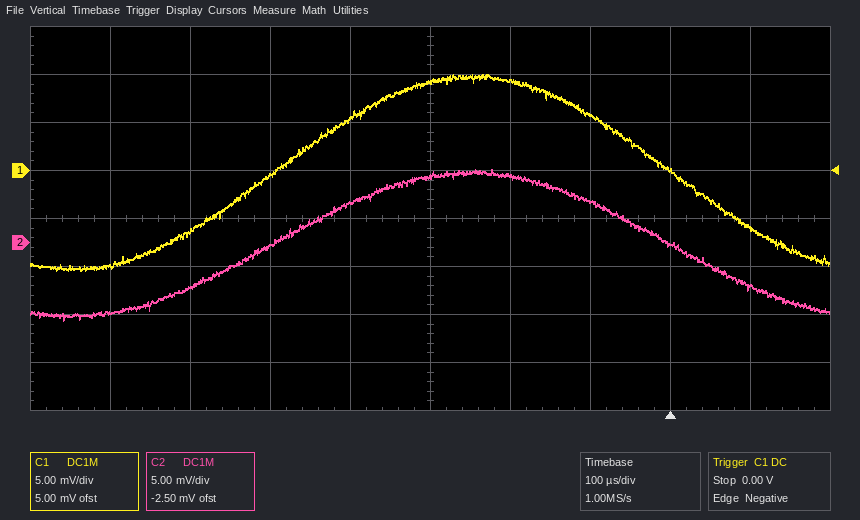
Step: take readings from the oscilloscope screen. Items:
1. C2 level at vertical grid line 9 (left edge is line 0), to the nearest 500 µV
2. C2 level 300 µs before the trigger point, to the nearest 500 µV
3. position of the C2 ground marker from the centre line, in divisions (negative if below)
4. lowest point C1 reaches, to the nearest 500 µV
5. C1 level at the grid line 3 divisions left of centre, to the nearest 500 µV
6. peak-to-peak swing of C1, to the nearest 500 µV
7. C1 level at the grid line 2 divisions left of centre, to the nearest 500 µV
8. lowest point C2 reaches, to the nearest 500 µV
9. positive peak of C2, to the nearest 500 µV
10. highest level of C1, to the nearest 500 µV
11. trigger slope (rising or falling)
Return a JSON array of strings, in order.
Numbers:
["-4.5 mV", "7.0 mV", "-0.5 div", "-10.5 mV", "-6.5 mV", "20.5 mV", "-500 µV", "-8.0 mV", "7.5 mV", "10.0 mV", "falling"]
